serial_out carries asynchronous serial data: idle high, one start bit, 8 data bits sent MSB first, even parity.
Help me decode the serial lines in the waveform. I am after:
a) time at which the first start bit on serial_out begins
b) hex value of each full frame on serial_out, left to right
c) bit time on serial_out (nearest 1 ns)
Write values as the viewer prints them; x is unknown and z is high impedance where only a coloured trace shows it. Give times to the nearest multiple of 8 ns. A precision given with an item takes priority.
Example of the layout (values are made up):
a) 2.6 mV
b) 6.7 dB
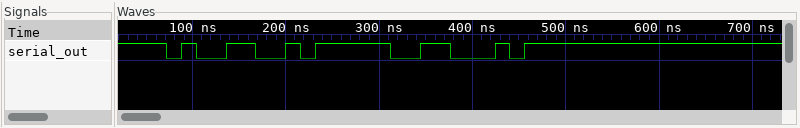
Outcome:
a) 72 ns
b) 99, 62
c) 16 ns
